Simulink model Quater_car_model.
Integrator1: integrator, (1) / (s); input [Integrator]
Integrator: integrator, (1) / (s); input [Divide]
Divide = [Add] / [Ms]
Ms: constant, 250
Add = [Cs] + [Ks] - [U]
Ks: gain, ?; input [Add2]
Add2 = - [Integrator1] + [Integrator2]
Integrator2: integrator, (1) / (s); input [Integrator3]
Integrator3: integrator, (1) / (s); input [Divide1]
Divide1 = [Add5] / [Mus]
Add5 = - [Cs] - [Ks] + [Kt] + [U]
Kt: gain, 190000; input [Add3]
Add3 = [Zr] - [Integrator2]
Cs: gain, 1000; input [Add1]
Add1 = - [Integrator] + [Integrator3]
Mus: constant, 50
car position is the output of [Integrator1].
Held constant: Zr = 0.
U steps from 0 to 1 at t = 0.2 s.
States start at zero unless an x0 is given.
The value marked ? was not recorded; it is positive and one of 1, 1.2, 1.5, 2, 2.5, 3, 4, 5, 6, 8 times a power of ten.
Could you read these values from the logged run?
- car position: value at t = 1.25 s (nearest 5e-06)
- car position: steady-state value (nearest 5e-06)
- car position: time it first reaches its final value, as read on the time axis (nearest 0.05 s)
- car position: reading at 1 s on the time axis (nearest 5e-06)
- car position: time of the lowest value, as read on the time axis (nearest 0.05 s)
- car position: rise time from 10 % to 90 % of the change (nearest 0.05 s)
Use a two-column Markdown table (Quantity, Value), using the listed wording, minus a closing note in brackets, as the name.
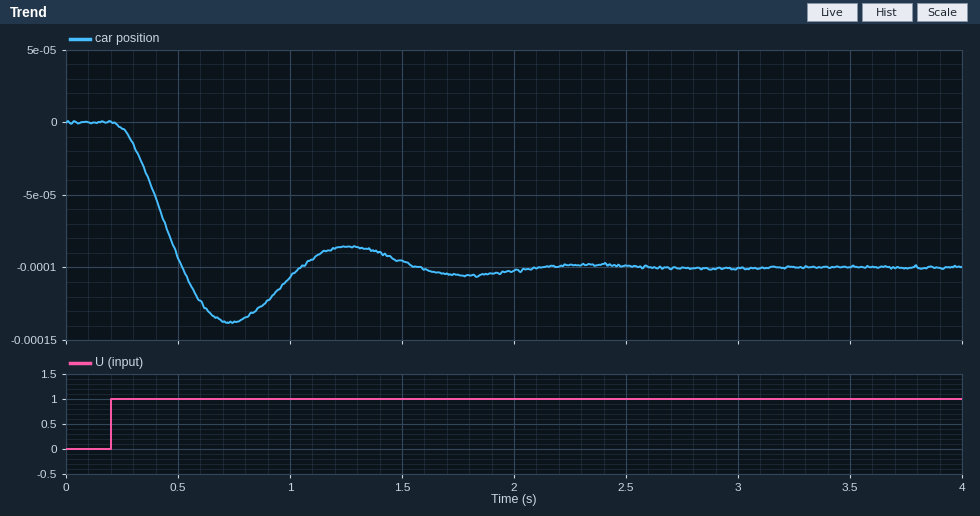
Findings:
| Quantity | Value |
|---|---|
| car position: value at t = 1.25 s | -0.000085 |
| car position: steady-state value | -0.000100 |
| car position: time it first reaches its final value, as read on the time axis | 0.50 s |
| car position: reading at 1 s on the time axis | -0.000105 |
| car position: time of the lowest value, as read on the time axis | 0.75 s |
| car position: rise time from 10 % to 90 % of the change | 0.20 s |
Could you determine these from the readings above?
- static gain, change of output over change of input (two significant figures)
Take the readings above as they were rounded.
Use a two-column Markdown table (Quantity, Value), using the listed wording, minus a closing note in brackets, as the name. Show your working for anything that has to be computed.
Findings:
| Quantity | Value |
|---|---|
| static gain, change of output over change of input | (-0.0001 - 0) / (1 - 0) = -0.00010 |
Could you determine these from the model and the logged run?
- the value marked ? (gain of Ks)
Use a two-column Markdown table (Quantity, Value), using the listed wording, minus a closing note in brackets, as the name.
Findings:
| Quantity | Value |
|---|---|
| the value marked ? | 10000 |
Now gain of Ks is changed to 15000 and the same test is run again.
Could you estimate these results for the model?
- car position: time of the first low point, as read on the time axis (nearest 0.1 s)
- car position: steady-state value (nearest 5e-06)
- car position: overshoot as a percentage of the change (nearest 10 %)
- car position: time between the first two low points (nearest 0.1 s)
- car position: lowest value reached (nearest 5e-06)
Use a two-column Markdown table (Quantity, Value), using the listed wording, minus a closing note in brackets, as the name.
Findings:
| Quantity | Value |
|---|---|
| car position: time of the first low point, as read on the time axis | 0.6 s |
| car position: steady-state value | -0.000065 |
| car position: overshoot as a percentage of the change | 50 % |
| car position: time between the first two low points | 0.9 s |
| car position: lowest value reached | -0.000100 |
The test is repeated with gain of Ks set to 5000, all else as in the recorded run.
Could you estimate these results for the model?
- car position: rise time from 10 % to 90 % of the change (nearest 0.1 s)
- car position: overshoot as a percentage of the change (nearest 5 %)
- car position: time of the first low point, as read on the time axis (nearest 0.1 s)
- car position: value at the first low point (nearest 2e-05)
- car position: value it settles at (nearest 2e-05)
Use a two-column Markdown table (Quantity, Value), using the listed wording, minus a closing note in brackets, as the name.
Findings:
| Quantity | Value |
|---|---|
| car position: rise time from 10 % to 90 % of the change | 0.3 s |
| car position: overshoot as a percentage of the change | 20 % |
| car position: time of the first low point, as read on the time axis | 1.0 s |
| car position: value at the first low point | -0.00024 |
| car position: value it settles at | -0.00020 |
